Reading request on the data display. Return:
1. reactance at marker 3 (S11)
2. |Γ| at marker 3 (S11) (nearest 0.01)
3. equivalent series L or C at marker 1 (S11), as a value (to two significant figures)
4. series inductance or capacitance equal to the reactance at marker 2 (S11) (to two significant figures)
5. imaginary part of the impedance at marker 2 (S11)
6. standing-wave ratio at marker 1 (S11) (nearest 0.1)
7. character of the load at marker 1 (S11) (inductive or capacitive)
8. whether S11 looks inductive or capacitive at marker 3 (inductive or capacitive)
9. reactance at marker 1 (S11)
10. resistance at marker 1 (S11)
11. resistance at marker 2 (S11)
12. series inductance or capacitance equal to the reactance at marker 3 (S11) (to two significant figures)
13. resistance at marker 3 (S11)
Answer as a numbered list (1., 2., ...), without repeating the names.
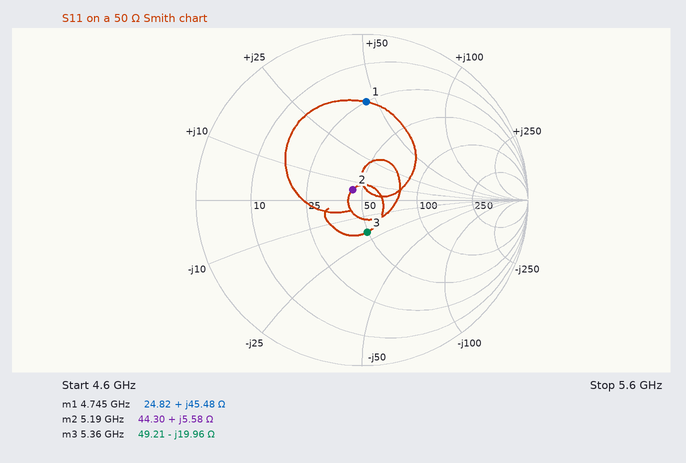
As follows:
1. -19.96 Ω
2. 0.20
3. 1.5 nH
4. 170 pH
5. +5.58 Ω
6. 3.9
7. inductive
8. capacitive
9. +45.48 Ω
10. 24.82 Ω
11. 44.30 Ω
12. 1.5 pF
13. 49.21 Ω
